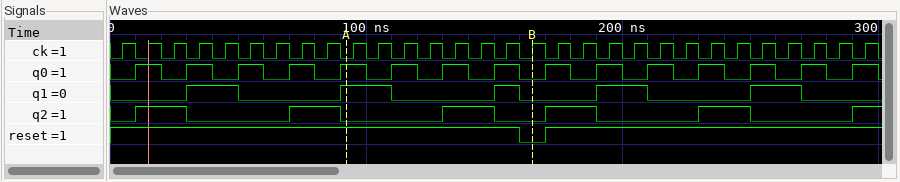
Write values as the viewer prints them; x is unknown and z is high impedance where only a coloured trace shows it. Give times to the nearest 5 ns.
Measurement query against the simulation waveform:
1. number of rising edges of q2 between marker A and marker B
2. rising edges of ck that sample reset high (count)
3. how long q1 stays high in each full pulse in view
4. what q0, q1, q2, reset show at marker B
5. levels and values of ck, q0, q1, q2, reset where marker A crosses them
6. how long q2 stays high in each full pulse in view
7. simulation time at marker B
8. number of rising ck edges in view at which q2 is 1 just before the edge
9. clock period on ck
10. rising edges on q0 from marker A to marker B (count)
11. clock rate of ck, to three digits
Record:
1
29
20 ns, 20 ns, 10 ns, 20 ns, 20 ns
q0=0, q1=0, q2=0, reset=0
ck=0, q0=1, q1=1, q2=0, reset=1
20 ns, 20 ns, 20 ns, 20 ns, 20 ns
165 ns
11
10 ns
3
100 MHz
